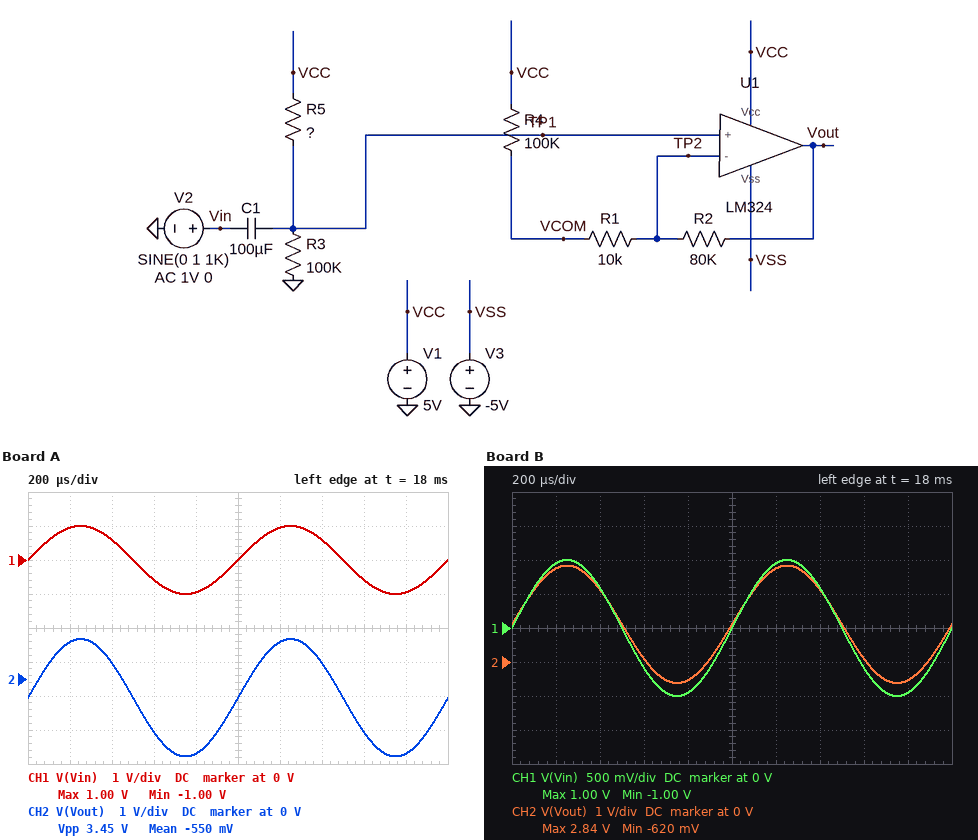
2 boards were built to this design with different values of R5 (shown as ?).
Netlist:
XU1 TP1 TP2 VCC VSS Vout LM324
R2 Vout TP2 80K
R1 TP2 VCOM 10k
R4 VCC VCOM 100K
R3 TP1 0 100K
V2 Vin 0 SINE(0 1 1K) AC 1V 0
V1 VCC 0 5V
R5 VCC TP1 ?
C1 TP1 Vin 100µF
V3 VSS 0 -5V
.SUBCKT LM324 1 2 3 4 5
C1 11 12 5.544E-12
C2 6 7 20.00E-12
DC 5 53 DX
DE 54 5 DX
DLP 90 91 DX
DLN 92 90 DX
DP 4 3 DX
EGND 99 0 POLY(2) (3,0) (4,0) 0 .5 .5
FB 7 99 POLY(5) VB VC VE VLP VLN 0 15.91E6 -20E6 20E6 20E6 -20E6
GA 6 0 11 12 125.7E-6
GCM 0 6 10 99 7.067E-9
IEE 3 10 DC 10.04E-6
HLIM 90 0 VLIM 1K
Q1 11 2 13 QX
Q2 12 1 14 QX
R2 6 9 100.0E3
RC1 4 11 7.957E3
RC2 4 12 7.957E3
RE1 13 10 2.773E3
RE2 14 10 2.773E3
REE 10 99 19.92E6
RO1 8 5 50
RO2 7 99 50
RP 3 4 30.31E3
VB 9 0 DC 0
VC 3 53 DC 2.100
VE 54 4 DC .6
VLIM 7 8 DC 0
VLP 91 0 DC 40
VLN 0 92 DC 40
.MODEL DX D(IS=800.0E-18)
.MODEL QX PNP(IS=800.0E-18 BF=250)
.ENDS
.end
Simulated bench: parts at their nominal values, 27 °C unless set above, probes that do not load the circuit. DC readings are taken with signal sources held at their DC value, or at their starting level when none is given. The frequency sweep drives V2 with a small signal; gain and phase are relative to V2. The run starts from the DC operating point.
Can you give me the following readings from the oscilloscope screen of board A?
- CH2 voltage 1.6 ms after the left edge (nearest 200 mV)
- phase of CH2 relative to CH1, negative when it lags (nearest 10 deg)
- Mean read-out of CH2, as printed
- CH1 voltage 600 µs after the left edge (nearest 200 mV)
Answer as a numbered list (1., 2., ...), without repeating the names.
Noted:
1. -1.6 V
2. 0 deg
3. -550 mV
4. -600 mV
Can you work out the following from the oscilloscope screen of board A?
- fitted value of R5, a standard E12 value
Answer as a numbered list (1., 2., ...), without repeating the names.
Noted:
1. 180 kΩ
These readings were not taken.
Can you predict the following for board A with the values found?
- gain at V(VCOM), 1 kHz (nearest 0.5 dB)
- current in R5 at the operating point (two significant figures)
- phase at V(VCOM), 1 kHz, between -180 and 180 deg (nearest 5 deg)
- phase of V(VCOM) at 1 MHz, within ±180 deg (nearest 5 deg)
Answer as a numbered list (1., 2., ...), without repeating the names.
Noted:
1. -1.0 dB
2. 18 µA
3. 0 deg
4. -90 deg
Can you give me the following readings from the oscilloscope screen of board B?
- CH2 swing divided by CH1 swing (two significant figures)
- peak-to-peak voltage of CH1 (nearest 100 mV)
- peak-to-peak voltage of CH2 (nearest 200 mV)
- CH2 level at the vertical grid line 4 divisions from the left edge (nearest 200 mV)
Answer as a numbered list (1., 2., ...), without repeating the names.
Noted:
1. 1.7
2. 2.0 V
3. 3.4 V
4. -600 mV
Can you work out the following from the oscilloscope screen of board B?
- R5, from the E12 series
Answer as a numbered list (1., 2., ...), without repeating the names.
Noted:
1. 82 kΩ
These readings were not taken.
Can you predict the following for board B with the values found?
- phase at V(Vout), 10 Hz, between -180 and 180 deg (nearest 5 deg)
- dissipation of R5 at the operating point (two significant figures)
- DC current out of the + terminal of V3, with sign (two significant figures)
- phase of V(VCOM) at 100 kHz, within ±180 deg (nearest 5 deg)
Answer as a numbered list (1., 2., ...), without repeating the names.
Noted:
1. 0 deg
2. 62 µW
3. -340 µA
4. -10 deg
